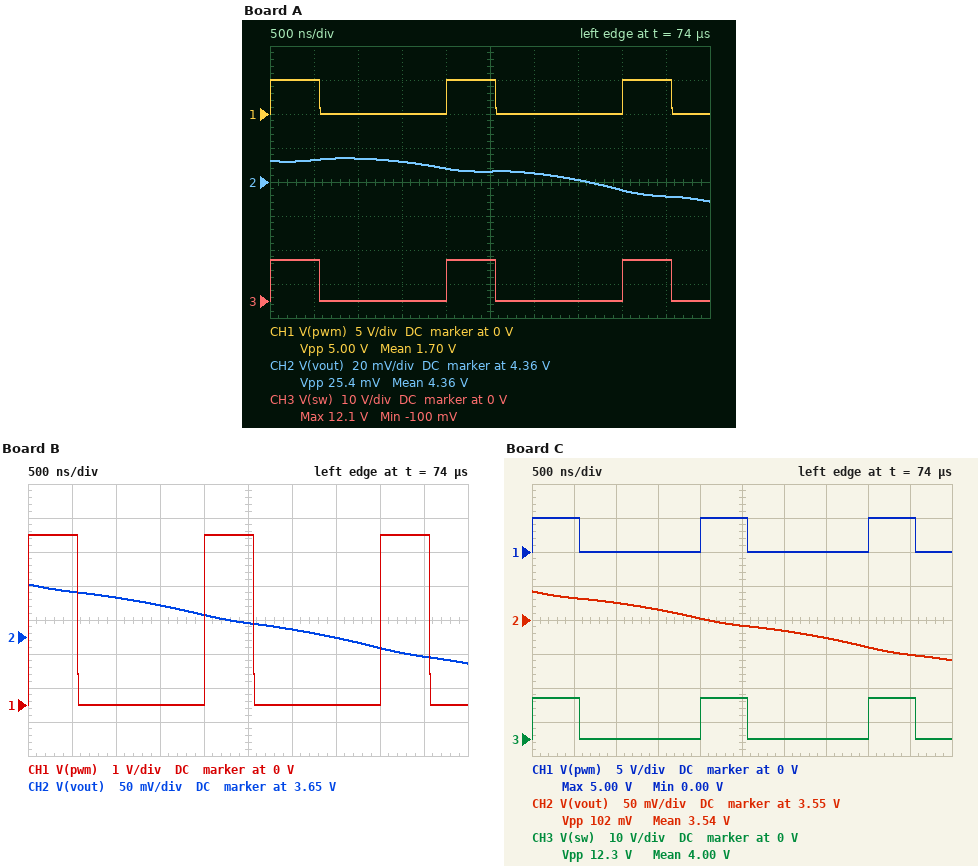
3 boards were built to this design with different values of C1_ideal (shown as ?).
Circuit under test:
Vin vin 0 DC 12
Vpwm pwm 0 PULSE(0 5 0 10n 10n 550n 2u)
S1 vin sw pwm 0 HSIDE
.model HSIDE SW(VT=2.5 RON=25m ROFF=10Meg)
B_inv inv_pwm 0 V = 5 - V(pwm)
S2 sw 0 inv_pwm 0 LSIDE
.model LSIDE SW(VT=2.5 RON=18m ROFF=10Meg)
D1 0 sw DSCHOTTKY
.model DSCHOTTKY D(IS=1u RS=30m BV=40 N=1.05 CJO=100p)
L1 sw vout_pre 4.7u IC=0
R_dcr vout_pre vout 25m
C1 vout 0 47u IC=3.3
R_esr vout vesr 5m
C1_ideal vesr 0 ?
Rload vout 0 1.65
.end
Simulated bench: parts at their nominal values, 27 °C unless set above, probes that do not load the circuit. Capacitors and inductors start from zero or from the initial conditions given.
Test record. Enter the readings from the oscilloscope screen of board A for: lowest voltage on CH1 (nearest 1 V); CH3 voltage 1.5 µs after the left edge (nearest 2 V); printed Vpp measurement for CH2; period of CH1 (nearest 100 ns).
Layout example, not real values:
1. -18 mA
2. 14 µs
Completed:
1. 0 V
2. 0 V
3. 25.4 mV
4. 2.0 µs
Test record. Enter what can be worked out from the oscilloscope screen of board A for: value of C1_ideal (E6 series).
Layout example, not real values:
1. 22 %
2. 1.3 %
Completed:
1. 68 µF
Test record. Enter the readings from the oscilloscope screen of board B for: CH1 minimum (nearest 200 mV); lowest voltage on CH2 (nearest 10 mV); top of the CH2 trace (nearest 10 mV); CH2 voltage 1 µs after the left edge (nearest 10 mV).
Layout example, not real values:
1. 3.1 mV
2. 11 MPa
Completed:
1. 0 V
2. 3.61 V
3. 3.73 V
4. 3.71 V
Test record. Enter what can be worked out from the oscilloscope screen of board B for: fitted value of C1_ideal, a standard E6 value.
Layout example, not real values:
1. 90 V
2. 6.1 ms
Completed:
1. 22 µF
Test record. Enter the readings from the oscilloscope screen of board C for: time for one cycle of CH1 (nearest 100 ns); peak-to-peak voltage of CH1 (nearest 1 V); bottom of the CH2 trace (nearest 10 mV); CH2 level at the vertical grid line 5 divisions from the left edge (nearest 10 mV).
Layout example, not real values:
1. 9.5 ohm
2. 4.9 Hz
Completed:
1. 2.0 µs
2. 5 V
3. 3.49 V
4. 3.54 V
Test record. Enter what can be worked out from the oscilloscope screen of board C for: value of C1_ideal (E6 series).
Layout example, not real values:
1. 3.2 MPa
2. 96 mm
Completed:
1. 15 µF
